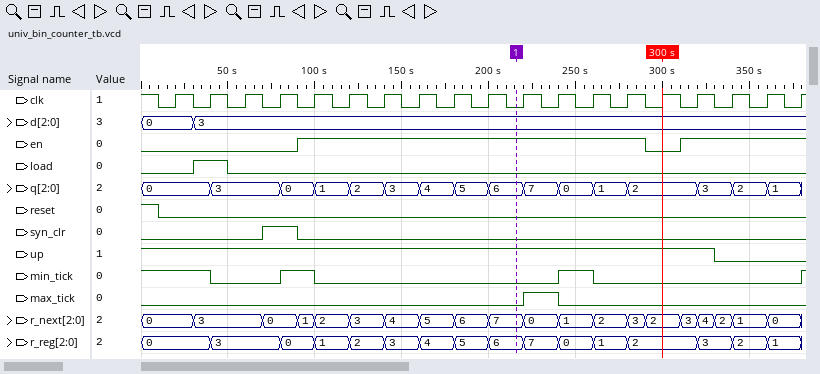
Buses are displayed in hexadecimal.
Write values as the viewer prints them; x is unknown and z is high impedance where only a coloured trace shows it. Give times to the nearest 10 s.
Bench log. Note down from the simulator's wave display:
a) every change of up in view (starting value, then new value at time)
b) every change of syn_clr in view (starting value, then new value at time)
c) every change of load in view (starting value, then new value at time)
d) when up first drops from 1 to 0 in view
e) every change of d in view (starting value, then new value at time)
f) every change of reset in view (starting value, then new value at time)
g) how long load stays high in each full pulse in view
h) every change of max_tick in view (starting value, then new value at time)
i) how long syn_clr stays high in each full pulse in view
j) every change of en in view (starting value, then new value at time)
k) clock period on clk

1, 0 at 330 s
0, 1 at 70 s, 0 at 90 s
0, 1 at 30 s, 0 at 50 s
330 s
0, 3 at 30 s
1, 0 at 10 s
20 s
0, 1 at 220 s, 0 at 240 s
20 s
0, 1 at 90 s, 0 at 290 s, 1 at 310 s
20 s
